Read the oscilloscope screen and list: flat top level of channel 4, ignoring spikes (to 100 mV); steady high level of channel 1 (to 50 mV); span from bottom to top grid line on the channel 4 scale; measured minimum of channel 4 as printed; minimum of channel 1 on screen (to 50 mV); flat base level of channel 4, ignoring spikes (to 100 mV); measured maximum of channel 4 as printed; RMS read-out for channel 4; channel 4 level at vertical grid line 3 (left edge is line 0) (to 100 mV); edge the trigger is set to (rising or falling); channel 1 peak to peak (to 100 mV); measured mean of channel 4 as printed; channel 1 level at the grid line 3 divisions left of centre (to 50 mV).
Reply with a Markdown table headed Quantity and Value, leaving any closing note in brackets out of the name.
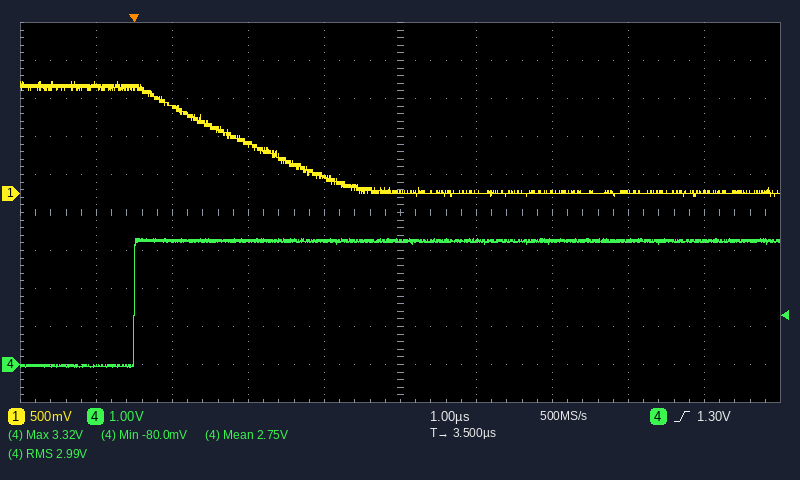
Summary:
| Quantity | Value |
|---|---|
| flat top level of channel 4, ignoring spikes | 3.2 V |
| steady high level of channel 1 | 1.40 V |
| span from bottom to top grid line on the channel 4 scale | 10 V |
| measured minimum of channel 4 as printed | -80.0 mV |
| minimum of channel 1 on screen | -50 mV |
| flat base level of channel 4, ignoring spikes | 0.0 V |
| measured maximum of channel 4 as printed | 3.32 V |
| RMS read-out for channel 4 | 2.99 V |
| channel 4 level at vertical grid line 3 (left edge is line 0) | 3.2 V |
| edge the trigger is set to | rising |
| channel 1 peak to peak | 1.50 V |
| measured mean of channel 4 as printed | 2.75 V |
| channel 1 level at the grid line 3 divisions left of centre | 1.15 V |
